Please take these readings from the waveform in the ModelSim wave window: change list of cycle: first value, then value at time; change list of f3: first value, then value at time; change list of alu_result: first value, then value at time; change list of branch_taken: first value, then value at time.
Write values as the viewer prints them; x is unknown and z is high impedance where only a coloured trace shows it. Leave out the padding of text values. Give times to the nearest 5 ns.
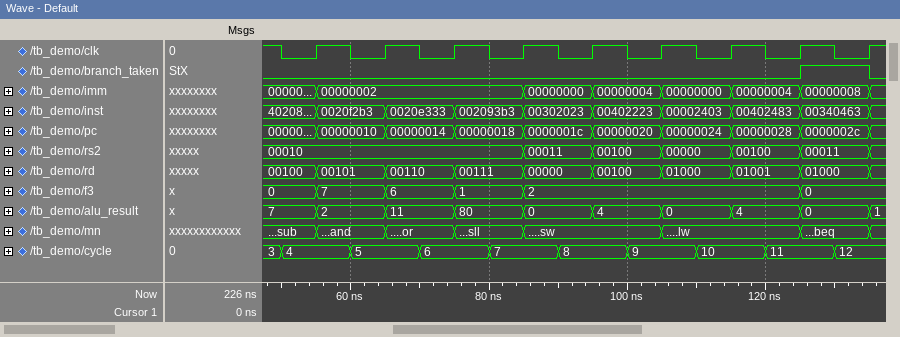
3, 4 at 50 ns, 5 at 60 ns, 6 at 70 ns, 7 at 80 ns, 8 at 90 ns, 9 at 100 ns, 10 at 110 ns, 11 at 120 ns, 12 at 130 ns
0, 7 at 55 ns, 6 at 65 ns, 1 at 75 ns, 2 at 85 ns, 0 at 125 ns
7, 2 at 55 ns, 11 at 65 ns, 80 at 75 ns, 0 at 85 ns, 4 at 95 ns, 0 at 105 ns, 4 at 115 ns, 0 at 125 ns, 1 at 135 ns
0, 1 at 125 ns, 0 at 135 ns
